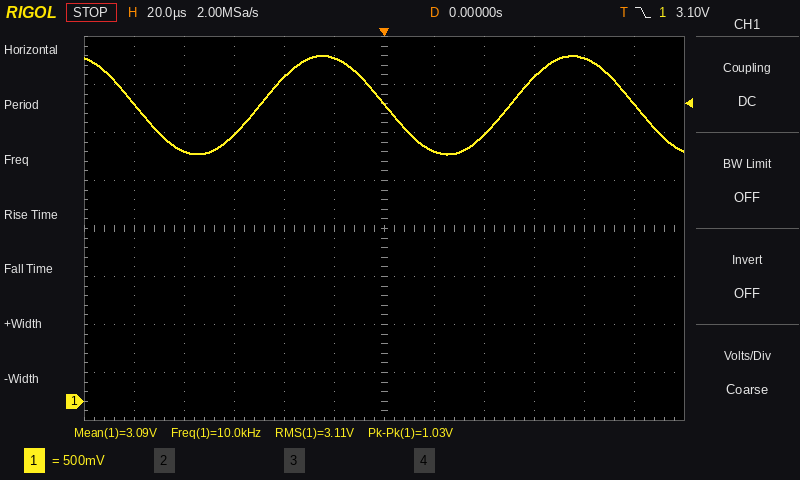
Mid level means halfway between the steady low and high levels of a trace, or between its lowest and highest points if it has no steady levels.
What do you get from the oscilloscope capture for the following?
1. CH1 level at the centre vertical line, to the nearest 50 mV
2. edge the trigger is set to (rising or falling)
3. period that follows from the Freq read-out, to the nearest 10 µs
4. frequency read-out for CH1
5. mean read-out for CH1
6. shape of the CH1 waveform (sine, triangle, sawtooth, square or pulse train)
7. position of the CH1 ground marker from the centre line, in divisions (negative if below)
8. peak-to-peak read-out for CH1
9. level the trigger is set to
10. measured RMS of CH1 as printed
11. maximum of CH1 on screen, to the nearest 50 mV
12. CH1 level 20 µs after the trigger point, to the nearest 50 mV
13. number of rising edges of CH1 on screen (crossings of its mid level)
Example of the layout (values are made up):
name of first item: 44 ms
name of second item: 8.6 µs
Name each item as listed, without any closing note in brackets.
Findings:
CH1 level at the centre vertical line, to the nearest 50 mV: 3.10 V
edge the trigger is set to: falling
period that follows from the Freq read-out, to the nearest 10 µs: 100 µs
frequency read-out for CH1: 10.0 kHz
mean read-out for CH1: 3.09 V
shape of the CH1 waveform: sine
position of the CH1 ground marker from the centre line, in divisions: -3.6 div
peak-to-peak read-out for CH1: 1.03 V
level the trigger is set to: 3.10 V
measured RMS of CH1 as printed: 3.11 V
maximum of CH1 on screen, to the nearest 50 mV: 3.60 V
CH1 level 20 µs after the trigger point, to the nearest 50 mV: 2.60 V
number of rising edges of CH1 on screen: 2
